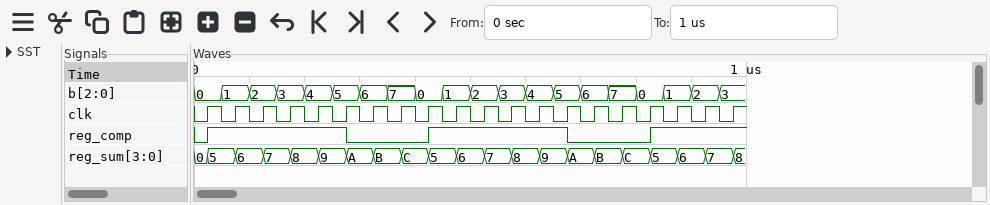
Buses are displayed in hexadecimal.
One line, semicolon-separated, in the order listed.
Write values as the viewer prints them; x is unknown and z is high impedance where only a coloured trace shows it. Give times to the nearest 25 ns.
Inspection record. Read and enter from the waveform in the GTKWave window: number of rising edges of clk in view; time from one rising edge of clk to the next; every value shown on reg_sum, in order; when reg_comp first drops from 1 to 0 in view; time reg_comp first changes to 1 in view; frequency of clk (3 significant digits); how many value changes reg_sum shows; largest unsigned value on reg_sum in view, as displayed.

20; 50 ns; 0, 5, 6, 7, 8, 9, A, B, C, 5, 6, 7, 8, 9, A, B, C, 5, 6, 7, 8; 275 ns; 25 ns; 20.0 MHz; 20; C
